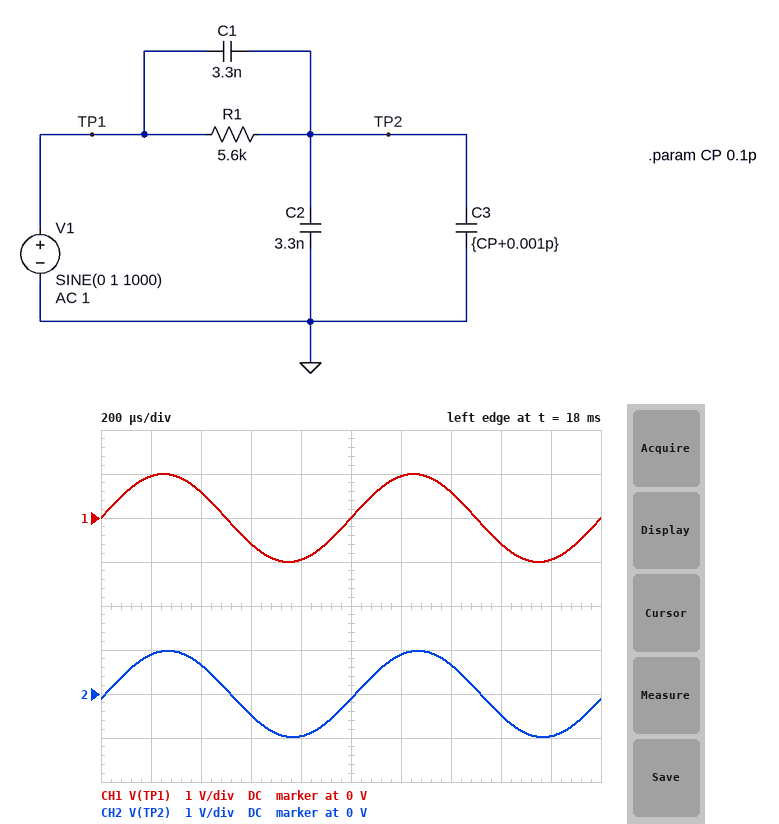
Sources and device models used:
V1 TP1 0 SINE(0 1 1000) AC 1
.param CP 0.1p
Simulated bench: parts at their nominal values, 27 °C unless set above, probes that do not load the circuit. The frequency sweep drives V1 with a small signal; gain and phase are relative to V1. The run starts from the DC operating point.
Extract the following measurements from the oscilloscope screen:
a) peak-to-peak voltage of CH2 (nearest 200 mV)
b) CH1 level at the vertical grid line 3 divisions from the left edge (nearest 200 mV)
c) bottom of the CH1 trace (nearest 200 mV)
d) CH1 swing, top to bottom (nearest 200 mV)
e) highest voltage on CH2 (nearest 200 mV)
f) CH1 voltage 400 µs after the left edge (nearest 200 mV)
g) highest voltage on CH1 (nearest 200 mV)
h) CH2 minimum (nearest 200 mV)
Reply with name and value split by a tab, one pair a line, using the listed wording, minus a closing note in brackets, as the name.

peak-to-peak voltage of CH2	2.0 V
CH1 level at the vertical grid line 3 divisions from the left edge	-600 mV
bottom of the CH1 trace	-1.0 V
CH1 swing, top to bottom	2.0 V
highest voltage on CH2	1.0 V
CH1 voltage 400 µs after the left edge	600 mV
highest voltage on CH1	1.0 V
CH2 minimum	-1.0 V
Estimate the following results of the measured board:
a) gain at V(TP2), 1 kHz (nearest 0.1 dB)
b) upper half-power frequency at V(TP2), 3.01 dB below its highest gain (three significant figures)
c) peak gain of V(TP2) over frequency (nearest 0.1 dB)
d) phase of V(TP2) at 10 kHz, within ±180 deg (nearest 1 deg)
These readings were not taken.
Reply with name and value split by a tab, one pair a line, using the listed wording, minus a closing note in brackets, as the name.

gain at V(TP2), 1 kHz	-0.2 dB
upper half-power frequency at V(TP2), 3.01 dB below its highest gain	6.09 kHz
peak gain of V(TP2) over frequency	0 dB
phase of V(TP2) at 10 kHz, within ±180 deg	-17 deg
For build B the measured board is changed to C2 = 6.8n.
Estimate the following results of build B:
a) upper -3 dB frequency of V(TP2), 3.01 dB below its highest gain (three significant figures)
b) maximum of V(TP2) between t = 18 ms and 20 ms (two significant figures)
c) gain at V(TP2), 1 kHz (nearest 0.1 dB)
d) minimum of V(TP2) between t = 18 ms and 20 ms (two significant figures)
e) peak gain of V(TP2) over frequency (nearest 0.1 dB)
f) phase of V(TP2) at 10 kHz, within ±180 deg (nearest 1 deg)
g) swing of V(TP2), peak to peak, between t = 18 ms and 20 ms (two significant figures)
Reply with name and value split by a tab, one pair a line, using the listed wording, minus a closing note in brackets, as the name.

upper -3 dB frequency of V(TP2), 3.01 dB below its highest gain	3.17 kHz
maximum of V(TP2) between t = 18 ms and 20 ms	950 mV
gain at V(TP2), 1 kHz	-0.5 dB
minimum of V(TP2) between t = 18 ms and 20 ms	-950 mV
peak gain of V(TP2) over frequency	0 dB
phase of V(TP2) at 10 kHz, within ±180 deg	-25 deg
swing of V(TP2), peak to peak, between t = 18 ms and 20 ms	1.9 V
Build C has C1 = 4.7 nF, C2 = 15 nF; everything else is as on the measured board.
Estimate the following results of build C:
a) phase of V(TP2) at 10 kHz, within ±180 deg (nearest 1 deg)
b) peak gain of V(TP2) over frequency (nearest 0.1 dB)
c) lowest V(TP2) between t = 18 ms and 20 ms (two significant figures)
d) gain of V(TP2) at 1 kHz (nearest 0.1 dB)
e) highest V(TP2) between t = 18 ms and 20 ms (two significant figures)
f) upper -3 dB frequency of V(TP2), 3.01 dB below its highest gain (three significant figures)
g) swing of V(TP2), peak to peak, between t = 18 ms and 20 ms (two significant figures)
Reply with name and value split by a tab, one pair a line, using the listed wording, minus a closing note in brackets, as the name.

phase of V(TP2) at 10 kHz, within ±180 deg	-23 deg
peak gain of V(TP2) over frequency	0 dB
lowest V(TP2) between t = 18 ms and 20 ms	-830 mV
gain of V(TP2) at 1 kHz	-1.6 dB
highest V(TP2) between t = 18 ms and 20 ms	830 mV
upper -3 dB frequency of V(TP2), 3.01 dB below its highest gain	1.53 kHz
swing of V(TP2), peak to peak, between t = 18 ms and 20 ms	1.7 V
